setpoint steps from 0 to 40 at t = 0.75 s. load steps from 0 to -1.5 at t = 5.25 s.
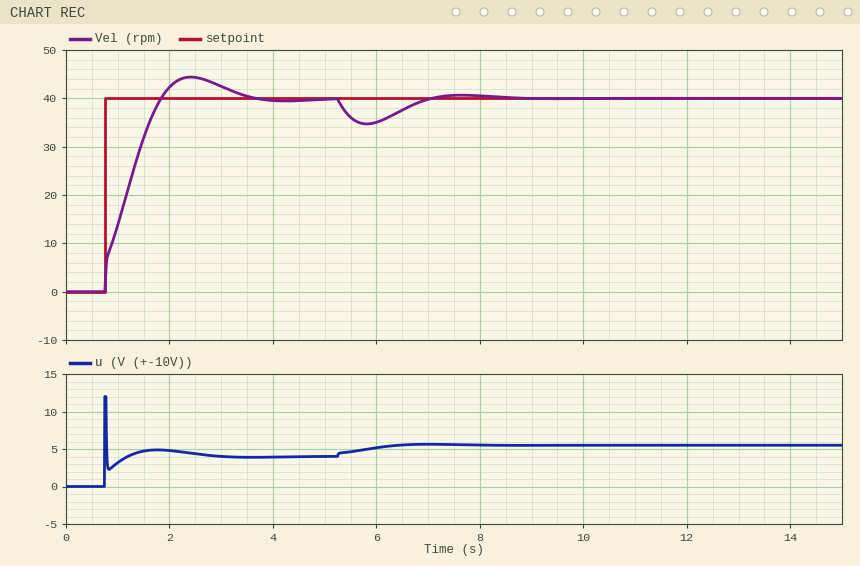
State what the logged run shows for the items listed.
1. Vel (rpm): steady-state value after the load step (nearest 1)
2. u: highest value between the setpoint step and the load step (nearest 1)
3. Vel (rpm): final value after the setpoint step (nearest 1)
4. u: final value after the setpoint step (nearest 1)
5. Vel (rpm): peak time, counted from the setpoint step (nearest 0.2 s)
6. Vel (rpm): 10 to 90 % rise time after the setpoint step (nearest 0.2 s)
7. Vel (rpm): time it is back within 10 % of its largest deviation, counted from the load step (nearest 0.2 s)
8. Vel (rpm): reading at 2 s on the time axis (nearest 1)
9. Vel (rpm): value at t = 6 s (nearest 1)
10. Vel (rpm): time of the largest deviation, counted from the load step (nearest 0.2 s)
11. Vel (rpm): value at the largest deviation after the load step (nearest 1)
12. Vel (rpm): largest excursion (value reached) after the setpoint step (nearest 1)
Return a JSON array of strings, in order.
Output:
["40", "12", "40", "4", "1.6 s", "0.8 s", "2.8 s", "42", "35", "0.6 s", "35", "44"]
